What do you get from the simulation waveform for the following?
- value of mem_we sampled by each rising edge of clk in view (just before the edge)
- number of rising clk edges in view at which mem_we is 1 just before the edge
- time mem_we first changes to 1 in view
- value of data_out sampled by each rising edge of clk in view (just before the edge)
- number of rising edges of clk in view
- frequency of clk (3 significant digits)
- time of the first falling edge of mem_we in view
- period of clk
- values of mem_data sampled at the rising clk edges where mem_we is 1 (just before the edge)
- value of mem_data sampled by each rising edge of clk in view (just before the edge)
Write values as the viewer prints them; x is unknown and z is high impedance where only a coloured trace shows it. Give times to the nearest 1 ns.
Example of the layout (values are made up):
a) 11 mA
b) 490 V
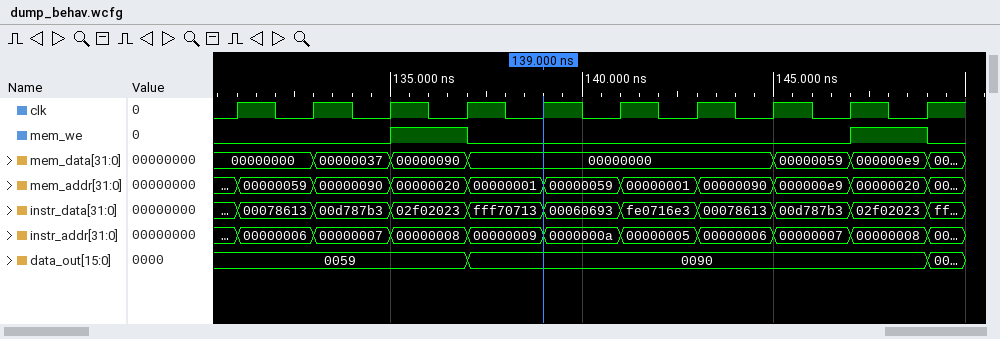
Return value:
a) 0 0 0 1 0 0 0 0 0 1
b) 2
c) 135 ns
d) 0059, 0059, 0059, 0059, 0090, 0090, 0090, 0090, 0090, 0090
e) 10
f) 500 MHz
g) 137 ns
h) 2 ns
i) 00000090, 000000e9
j) 00000000, 00000000, 00000037, 00000090, 00000000, 00000000, 00000000, 00000000, 00000059, 000000e9
